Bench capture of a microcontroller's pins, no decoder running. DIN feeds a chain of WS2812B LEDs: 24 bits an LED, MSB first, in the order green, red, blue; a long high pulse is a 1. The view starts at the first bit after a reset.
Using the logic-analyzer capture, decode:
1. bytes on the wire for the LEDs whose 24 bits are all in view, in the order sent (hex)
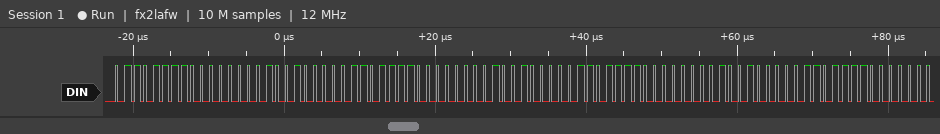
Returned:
6F 00 90 6F 00 90 6F 00 90
